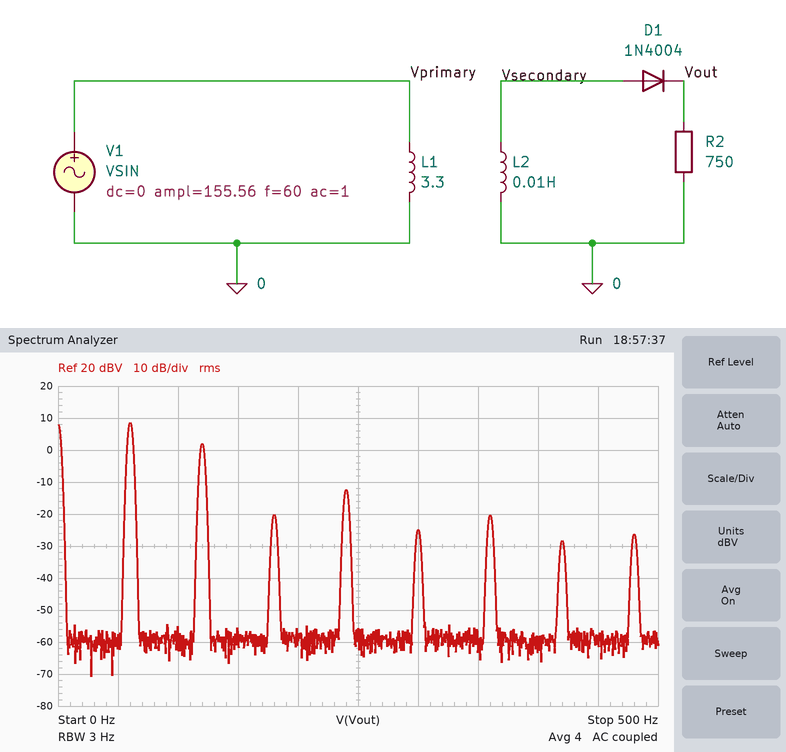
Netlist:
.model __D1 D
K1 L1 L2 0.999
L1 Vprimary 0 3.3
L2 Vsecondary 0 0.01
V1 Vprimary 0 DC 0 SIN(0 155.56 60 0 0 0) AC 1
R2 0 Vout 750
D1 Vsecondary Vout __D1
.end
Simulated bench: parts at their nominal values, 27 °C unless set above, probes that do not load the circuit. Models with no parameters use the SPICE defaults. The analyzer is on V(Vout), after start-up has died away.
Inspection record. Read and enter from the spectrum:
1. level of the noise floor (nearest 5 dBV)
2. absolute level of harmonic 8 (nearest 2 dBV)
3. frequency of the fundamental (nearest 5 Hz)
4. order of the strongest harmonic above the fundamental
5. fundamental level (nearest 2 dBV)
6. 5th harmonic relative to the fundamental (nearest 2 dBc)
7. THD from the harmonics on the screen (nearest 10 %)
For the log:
-60 dBV
-26 dBV
60 Hz
2
8 dBV
-34 dBc
50 %
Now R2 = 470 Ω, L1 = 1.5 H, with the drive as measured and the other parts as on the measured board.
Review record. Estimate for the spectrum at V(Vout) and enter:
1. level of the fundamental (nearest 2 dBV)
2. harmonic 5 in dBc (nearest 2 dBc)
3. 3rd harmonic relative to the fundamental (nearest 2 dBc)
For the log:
12 dBV
-36 dBc
-32 dBc
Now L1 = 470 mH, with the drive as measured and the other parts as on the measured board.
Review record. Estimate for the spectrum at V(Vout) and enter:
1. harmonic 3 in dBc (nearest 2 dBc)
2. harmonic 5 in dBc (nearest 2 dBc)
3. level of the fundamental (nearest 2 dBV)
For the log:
-38 dBc
-42 dBc
18 dBV
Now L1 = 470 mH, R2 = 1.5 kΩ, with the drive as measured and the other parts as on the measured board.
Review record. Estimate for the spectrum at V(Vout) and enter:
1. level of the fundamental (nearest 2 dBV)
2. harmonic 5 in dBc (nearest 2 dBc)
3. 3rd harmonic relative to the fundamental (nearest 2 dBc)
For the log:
18 dBV
-42 dBc
-38 dBc
